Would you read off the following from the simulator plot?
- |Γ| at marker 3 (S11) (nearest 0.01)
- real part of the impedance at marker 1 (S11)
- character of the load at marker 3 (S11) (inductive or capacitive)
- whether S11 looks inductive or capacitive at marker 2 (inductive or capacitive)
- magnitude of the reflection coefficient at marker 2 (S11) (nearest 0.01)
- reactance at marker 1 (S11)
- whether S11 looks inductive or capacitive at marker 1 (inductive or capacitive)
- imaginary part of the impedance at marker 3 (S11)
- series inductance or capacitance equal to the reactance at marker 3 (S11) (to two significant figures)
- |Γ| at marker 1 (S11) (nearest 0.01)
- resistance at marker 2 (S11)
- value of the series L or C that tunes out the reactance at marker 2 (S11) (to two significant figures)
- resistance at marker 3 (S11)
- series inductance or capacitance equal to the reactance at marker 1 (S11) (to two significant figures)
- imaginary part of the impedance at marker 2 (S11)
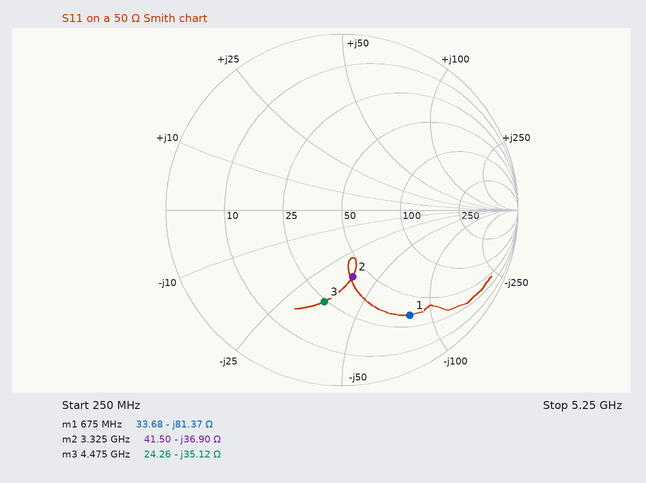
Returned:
0.53
33.68 Ω
capacitive
capacitive
0.38
-81.37 Ω
capacitive
-35.12 Ω
1.0 pF
0.71
41.50 Ω
1.8 nH
24.26 Ω
2.9 pF
-36.90 Ω
